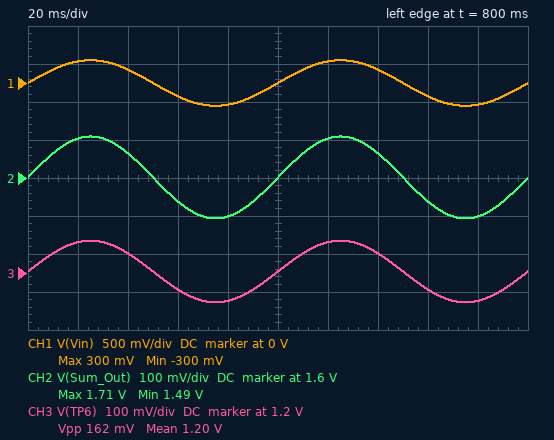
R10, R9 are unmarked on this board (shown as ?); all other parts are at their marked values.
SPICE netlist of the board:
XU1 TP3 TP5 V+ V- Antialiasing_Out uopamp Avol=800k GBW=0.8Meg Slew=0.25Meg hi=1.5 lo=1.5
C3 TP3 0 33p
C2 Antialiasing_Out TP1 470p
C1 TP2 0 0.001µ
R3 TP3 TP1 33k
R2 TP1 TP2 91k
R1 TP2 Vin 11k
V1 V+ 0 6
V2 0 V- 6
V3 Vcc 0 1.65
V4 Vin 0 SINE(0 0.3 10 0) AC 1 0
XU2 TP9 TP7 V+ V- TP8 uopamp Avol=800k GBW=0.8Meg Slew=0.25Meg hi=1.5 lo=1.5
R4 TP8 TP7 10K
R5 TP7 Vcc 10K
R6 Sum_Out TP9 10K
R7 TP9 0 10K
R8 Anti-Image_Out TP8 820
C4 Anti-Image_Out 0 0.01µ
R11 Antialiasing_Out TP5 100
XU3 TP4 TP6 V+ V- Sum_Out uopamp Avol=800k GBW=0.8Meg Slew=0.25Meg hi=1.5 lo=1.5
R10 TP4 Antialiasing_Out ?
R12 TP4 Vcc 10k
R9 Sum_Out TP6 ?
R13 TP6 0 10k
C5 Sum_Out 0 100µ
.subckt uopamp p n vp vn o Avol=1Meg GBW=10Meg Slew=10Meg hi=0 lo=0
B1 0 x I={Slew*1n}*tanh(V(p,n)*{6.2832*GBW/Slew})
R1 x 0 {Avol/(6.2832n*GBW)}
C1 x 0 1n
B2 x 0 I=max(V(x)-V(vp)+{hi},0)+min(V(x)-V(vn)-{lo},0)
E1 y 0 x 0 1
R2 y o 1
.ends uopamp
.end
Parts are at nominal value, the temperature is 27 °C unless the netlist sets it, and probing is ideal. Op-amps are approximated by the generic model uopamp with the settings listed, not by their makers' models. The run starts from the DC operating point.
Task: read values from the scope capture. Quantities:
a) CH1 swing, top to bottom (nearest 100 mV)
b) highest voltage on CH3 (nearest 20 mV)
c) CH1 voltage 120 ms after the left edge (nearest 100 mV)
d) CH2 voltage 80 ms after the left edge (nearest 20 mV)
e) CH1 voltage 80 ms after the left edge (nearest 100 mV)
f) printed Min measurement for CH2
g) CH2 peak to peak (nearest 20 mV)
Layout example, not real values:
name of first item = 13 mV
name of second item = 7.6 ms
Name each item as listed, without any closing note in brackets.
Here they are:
CH1 swing, top to bottom = 600 mV
highest voltage on CH3 = 1.28 V
CH1 voltage 120 ms after the left edge = 300 mV
CH2 voltage 80 ms after the left edge = 1.50 V
CH1 voltage 80 ms after the left edge = -300 mV
printed Min measurement for CH2 = 1.49 V
CH2 peak to peak = 220 mV
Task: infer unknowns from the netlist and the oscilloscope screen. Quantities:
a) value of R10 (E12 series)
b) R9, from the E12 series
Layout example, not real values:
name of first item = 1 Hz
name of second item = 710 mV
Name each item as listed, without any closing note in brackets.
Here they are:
value of R10 = 27 kΩ
R9, from the E12 series = 3.3 kΩ
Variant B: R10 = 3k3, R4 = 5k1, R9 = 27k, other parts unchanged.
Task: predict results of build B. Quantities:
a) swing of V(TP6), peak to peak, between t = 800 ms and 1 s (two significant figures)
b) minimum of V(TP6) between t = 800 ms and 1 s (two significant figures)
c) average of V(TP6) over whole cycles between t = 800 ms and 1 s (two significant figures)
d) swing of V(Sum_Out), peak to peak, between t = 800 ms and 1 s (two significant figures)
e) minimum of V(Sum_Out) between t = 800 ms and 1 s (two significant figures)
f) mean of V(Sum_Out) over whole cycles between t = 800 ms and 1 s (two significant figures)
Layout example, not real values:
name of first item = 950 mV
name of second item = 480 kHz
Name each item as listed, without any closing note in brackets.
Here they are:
swing of V(TP6), peak to peak, between t = 800 ms and 1 s = 450 mV
minimum of V(TP6) between t = 800 ms and 1 s = 180 mV
average of V(TP6) over whole cycles between t = 800 ms and 1 s = 410 mV
swing of V(Sum_Out), peak to peak, between t = 800 ms and 1 s = 1.7 V
minimum of V(Sum_Out) between t = 800 ms and 1 s = 680 mV
mean of V(Sum_Out) over whole cycles between t = 800 ms and 1 s = 1.5 V
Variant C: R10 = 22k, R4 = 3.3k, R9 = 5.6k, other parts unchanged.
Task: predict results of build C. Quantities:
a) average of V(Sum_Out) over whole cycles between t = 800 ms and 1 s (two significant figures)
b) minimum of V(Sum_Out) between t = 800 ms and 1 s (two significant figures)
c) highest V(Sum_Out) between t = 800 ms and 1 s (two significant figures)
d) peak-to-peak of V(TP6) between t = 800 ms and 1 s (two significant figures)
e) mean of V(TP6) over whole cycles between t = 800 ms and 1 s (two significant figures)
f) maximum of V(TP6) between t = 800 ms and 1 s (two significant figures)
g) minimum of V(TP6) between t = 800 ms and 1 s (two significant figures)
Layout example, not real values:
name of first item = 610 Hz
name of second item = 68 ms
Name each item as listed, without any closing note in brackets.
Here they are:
average of V(Sum_Out) over whole cycles between t = 800 ms and 1 s = 1.8 V
minimum of V(Sum_Out) between t = 800 ms and 1 s = 1.6 V
highest V(Sum_Out) between t = 800 ms and 1 s = 1.9 V
peak-to-peak of V(TP6) between t = 800 ms and 1 s = 190 mV
mean of V(TP6) over whole cycles between t = 800 ms and 1 s = 1.1 V
maximum of V(TP6) between t = 800 ms and 1 s = 1.2 V
minimum of V(TP6) between t = 800 ms and 1 s = 1.0 V
